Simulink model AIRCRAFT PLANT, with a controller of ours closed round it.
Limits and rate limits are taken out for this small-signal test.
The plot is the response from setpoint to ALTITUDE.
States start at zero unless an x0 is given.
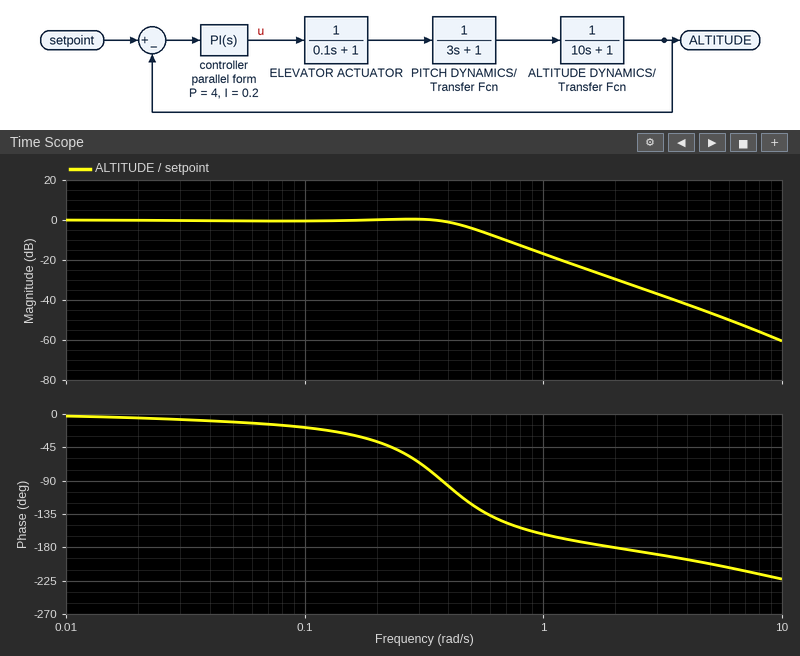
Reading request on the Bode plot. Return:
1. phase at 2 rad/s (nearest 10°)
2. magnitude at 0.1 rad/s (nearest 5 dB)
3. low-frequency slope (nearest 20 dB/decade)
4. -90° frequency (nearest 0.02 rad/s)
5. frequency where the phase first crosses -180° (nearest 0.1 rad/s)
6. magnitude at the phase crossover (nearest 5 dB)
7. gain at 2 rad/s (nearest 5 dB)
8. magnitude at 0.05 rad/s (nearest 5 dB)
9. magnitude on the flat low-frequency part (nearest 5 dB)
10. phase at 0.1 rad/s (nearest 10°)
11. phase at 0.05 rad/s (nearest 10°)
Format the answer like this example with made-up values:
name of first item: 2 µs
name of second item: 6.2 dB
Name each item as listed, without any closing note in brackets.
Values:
phase at 2 rad/s: -180°
magnitude at 0.1 rad/s: 0 dB
low-frequency slope: 0 dB/decade
-90° frequency: 0.38 rad/s
frequency where the phase first crosses -180°: 2.0 rad/s
magnitude at the phase crossover: -30 dB
gain at 2 rad/s: -30 dB
magnitude at 0.05 rad/s: 0 dB
magnitude on the flat low-frequency part: 0 dB
phase at 0.1 rad/s: -20°
phase at 0.05 rad/s: -10°
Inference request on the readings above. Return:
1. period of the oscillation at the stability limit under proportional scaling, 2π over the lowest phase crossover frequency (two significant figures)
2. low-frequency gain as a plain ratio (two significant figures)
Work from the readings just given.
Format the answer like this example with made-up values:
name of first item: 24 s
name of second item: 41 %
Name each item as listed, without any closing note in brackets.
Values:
period of the oscillation at the stability limit under proportional scaling, 2π over the lowest phase crossover frequency: 3.1 s
low-frequency gain as a plain ratio: 1.0
